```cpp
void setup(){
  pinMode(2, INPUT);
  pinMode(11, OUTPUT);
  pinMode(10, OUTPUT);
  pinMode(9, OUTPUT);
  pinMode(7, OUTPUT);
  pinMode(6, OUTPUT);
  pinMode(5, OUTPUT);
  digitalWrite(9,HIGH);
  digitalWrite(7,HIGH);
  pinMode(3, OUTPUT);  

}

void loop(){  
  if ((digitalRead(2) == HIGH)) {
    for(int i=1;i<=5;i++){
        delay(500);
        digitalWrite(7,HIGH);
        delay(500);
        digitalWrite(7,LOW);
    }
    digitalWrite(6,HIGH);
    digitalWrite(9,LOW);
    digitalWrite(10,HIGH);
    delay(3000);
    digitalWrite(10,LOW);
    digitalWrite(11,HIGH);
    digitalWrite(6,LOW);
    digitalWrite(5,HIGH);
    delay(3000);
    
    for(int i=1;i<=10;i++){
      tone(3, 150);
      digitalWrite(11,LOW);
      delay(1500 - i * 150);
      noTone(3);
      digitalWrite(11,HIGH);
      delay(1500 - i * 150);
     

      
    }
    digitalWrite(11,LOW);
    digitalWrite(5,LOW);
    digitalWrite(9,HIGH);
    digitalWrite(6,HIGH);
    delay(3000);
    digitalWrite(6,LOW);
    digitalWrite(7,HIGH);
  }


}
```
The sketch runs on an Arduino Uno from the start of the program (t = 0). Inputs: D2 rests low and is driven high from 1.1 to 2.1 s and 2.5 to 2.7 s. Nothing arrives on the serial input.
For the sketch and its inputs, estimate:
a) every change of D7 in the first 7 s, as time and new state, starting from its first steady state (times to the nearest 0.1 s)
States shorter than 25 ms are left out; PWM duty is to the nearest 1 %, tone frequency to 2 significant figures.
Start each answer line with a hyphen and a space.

- 0 s high; 2.1 s low; 2.6 s high; 3.1 s low; 3.6 s high; 4.1 s low; 4.6 s high; 5.1 s low; 5.6 s high; 6.1 s low
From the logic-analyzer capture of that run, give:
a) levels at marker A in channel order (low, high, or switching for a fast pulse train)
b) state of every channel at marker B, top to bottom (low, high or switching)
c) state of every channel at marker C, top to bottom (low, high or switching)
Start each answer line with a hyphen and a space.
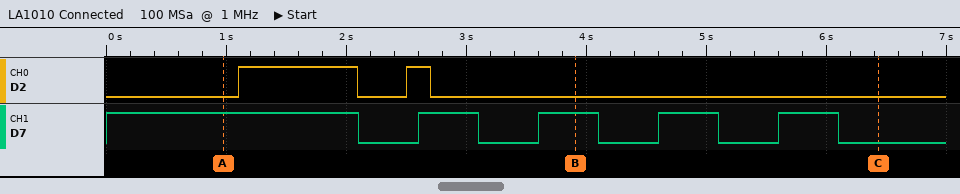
- D2 low, D7 high
- D2 low, D7 high
- D2 low, D7 low
